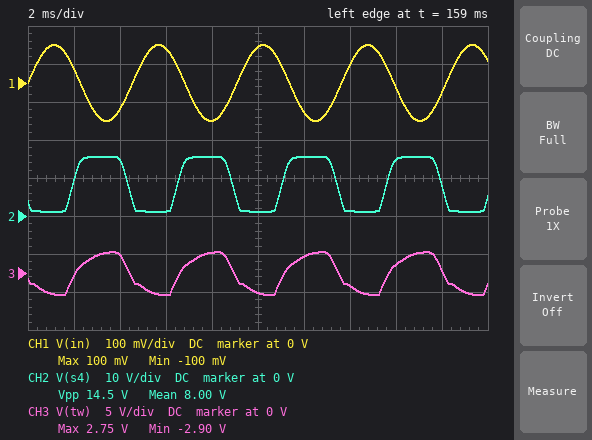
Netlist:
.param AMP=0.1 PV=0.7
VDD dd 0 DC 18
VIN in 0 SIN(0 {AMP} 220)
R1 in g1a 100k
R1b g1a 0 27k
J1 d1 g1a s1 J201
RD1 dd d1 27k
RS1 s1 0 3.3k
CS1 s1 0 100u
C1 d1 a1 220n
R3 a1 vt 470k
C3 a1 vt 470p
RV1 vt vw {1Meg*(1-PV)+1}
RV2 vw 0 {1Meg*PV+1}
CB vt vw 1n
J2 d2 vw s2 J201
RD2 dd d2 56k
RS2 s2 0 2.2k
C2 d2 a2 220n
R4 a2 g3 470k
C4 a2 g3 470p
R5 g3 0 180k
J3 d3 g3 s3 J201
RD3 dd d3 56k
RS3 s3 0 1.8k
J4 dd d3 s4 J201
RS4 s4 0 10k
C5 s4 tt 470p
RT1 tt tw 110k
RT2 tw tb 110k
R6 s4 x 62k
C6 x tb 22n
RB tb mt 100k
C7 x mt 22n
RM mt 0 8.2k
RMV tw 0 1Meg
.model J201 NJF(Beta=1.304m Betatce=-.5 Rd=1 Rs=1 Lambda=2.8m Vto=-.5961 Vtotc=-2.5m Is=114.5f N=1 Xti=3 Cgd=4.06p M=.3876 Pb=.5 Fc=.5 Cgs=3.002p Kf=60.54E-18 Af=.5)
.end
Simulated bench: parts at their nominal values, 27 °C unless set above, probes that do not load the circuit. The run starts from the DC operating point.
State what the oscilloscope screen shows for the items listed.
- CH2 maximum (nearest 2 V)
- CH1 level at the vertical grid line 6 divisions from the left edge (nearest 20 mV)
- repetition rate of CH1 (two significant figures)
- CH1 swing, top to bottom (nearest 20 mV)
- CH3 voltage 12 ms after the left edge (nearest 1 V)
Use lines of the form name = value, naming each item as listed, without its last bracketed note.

CH2 maximum = 16 V
CH1 level at the vertical grid line 6 divisions from the left edge = -80 mV
repetition rate of CH1 = 220 Hz
CH1 swing, top to bottom = 200 mV
CH3 voltage 12 ms after the left edge = 2 V
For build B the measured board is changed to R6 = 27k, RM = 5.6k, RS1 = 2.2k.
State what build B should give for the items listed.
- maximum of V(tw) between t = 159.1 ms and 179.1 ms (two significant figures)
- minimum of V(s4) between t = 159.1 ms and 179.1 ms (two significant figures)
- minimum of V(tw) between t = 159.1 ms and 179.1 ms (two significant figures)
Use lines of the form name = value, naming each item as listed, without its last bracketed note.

maximum of V(tw) between t = 159.1 ms and 179.1 ms = 4.1 V
minimum of V(s4) between t = 159.1 ms and 179.1 ms = 1.2 V
minimum of V(tw) between t = 159.1 ms and 179.1 ms = -4.4 V
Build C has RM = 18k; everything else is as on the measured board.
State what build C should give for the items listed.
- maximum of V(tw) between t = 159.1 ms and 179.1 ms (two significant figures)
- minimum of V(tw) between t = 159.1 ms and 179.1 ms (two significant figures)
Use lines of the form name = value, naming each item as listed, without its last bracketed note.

maximum of V(tw) between t = 159.1 ms and 179.1 ms = 3.0 V
minimum of V(tw) between t = 159.1 ms and 179.1 ms = -3.2 V
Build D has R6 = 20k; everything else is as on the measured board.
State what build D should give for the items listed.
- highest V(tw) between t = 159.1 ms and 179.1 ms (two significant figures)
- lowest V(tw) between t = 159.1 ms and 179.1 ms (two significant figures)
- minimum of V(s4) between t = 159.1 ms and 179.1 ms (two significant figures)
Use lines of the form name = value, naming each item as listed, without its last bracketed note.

highest V(tw) between t = 159.1 ms and 179.1 ms = 4.6 V
lowest V(tw) between t = 159.1 ms and 179.1 ms = -5.0 V
minimum of V(s4) between t = 159.1 ms and 179.1 ms = 1.2 V
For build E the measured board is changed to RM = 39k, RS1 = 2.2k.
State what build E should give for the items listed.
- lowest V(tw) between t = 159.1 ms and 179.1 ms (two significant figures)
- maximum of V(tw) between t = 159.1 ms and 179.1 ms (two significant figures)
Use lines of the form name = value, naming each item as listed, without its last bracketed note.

lowest V(tw) between t = 159.1 ms and 179.1 ms = -3.6 V
maximum of V(tw) between t = 159.1 ms and 179.1 ms = 3.4 V
